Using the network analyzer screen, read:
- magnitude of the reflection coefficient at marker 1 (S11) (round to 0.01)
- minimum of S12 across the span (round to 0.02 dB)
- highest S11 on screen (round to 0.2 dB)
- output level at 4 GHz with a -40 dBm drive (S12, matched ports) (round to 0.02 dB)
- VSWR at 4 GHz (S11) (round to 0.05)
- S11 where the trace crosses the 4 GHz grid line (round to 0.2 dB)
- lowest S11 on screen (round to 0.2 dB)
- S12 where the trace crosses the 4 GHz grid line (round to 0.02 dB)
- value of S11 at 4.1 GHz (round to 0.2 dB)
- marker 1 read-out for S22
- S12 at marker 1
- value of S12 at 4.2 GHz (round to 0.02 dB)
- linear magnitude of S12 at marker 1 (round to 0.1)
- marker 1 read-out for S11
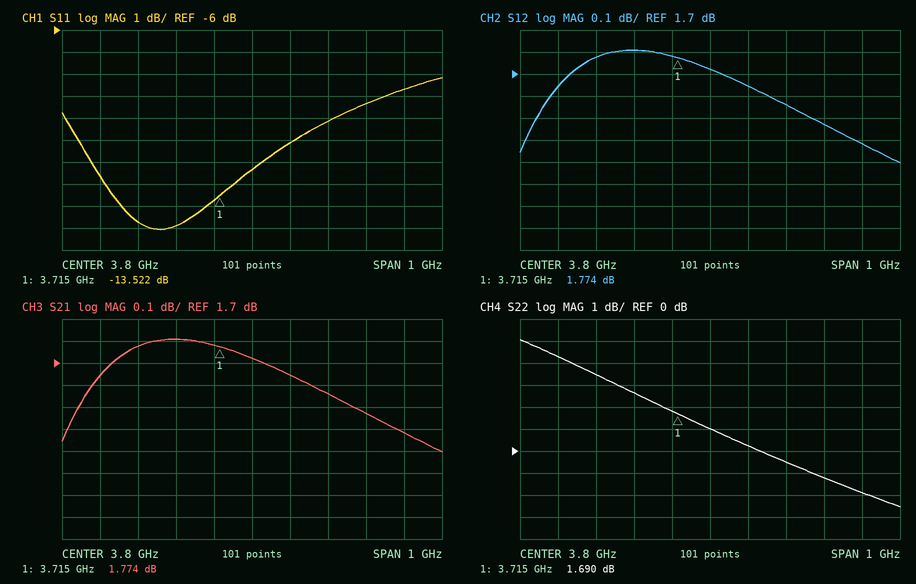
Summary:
0.21
1.30 dB
-8.2 dB
-38.44 dBm
1.90
-10.2 dB
-15.0 dB
1.56 dB
-9.4 dB
1.690 dB
1.774 dB
1.38 dB
1.2
-13.522 dB
